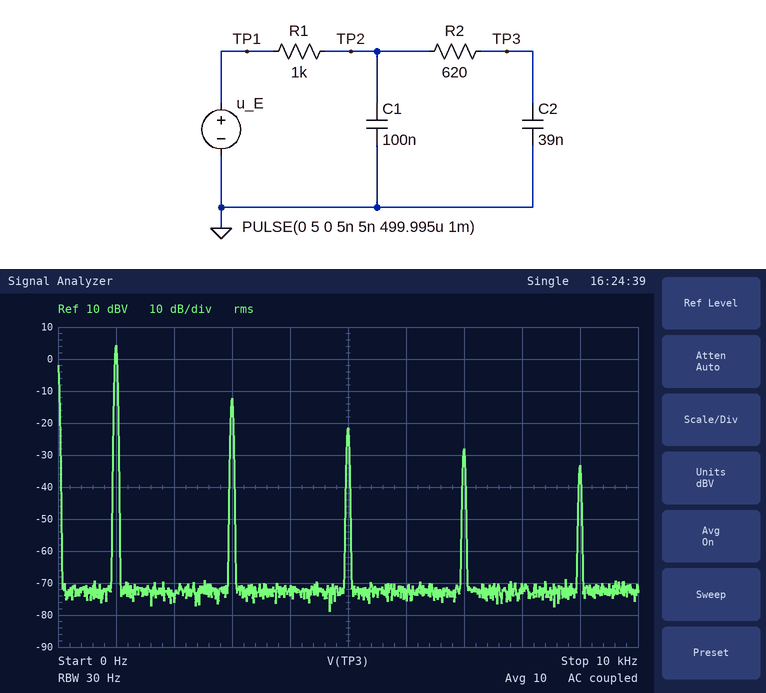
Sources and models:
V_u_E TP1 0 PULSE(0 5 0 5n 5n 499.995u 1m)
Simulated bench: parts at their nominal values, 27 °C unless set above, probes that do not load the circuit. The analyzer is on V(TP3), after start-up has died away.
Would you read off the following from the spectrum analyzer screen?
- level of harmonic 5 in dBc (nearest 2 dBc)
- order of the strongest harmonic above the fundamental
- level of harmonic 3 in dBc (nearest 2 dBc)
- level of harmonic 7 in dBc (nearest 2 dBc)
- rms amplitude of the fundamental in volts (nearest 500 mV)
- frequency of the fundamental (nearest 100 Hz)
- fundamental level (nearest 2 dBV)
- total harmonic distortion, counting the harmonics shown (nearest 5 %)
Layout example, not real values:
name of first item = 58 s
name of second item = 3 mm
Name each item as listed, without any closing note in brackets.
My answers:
level of harmonic 5 in dBc = -26 dBc
order of the strongest harmonic above the fundamental = 3
level of harmonic 3 in dBc = -16 dBc
level of harmonic 7 in dBc = -32 dBc
rms amplitude of the fundamental in volts = 1.5 V
frequency of the fundamental = 1.0 kHz
fundamental level = 4 dBV
total harmonic distortion, counting the harmonics shown = 15 %
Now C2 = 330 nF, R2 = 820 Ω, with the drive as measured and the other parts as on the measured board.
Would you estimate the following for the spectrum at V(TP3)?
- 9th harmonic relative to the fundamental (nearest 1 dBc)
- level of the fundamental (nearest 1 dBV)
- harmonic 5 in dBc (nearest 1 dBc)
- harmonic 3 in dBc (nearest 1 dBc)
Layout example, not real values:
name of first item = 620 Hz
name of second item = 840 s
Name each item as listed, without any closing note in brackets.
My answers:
9th harmonic relative to the fundamental = -46 dBc
level of the fundamental = -6 dBV
harmonic 5 in dBc = -32 dBc
harmonic 3 in dBc = -21 dBc
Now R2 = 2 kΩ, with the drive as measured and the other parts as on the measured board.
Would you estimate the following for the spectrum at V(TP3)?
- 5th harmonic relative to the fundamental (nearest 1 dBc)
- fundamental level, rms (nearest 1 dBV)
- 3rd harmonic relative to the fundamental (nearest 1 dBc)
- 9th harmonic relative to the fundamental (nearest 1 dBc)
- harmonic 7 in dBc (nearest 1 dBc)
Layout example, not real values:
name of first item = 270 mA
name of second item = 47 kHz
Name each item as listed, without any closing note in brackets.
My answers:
5th harmonic relative to the fundamental = -30 dBc
fundamental level, rms = 3 dBV
3rd harmonic relative to the fundamental = -19 dBc
9th harmonic relative to the fundamental = -44 dBc
harmonic 7 in dBc = -38 dBc
